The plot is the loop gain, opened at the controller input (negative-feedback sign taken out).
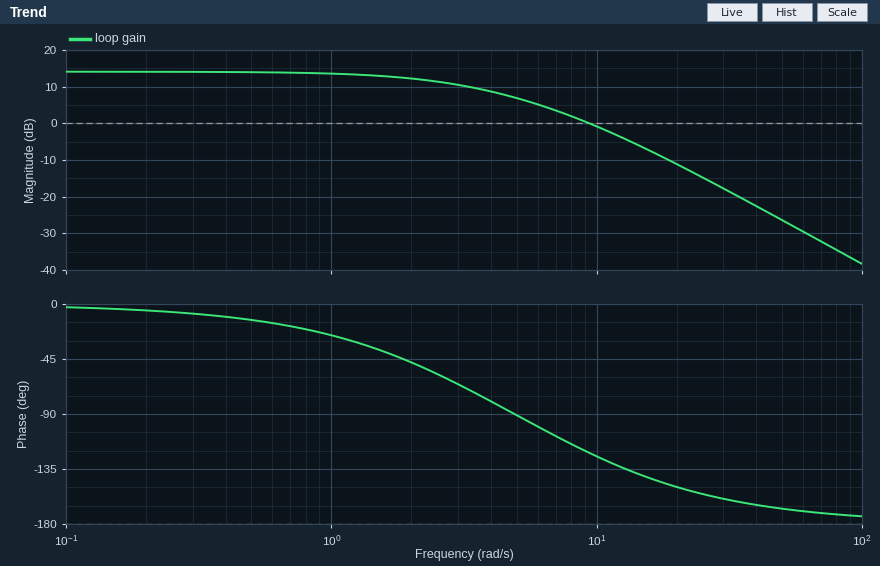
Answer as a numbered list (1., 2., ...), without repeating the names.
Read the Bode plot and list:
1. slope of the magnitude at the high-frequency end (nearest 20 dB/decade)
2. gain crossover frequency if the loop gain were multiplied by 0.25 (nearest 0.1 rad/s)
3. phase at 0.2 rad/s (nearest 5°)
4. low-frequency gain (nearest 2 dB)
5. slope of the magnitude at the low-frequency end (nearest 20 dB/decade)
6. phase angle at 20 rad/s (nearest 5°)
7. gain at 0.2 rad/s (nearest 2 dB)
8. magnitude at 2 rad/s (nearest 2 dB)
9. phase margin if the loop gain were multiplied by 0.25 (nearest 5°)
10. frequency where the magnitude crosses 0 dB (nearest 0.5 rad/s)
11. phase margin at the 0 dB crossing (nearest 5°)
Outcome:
1. -40 dB/decade
2. 2.1 rad/s
3. -5°
4. 14 dB
5. 0 dB/decade
6. -150°
7. 14 dB
8. 12 dB
9. 130°
10. 9.5 rad/s
11. 60°
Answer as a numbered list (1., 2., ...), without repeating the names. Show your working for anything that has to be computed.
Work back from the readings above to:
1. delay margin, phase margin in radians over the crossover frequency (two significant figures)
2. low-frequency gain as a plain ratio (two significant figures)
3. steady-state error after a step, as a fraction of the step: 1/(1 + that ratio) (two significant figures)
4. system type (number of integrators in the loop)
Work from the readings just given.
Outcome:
1. 60 × π / 180 / 9.5 = 0.11 s
2. 10^(14 / 20) = 5.0
3. 1 / (1 + 5) = 0.17
4. 0
